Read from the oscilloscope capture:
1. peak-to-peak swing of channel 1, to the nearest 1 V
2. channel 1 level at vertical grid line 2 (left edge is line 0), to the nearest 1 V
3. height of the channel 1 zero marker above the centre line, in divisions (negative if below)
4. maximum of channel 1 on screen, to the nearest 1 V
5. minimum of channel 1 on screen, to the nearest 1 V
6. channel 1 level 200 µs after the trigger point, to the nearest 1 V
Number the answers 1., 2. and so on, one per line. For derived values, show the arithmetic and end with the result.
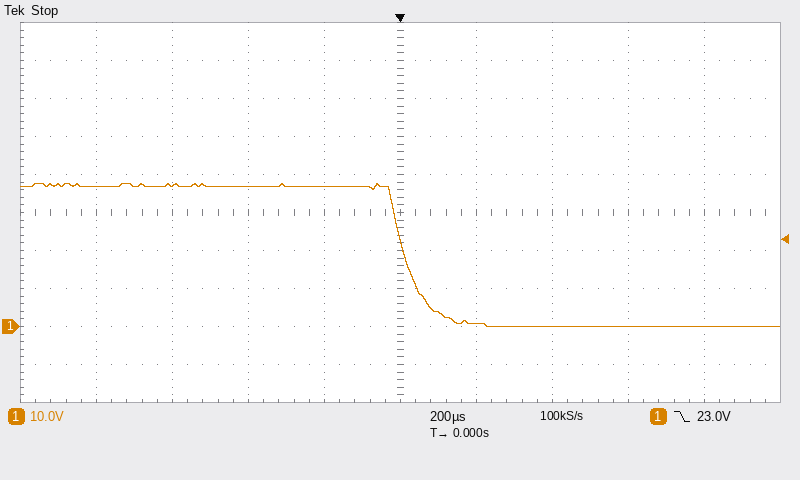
1. 38 V − (0 V) = 38 V
2. 37 V
3. -3.0 div
4. 38 V
5. 0 V
6. 1 V
